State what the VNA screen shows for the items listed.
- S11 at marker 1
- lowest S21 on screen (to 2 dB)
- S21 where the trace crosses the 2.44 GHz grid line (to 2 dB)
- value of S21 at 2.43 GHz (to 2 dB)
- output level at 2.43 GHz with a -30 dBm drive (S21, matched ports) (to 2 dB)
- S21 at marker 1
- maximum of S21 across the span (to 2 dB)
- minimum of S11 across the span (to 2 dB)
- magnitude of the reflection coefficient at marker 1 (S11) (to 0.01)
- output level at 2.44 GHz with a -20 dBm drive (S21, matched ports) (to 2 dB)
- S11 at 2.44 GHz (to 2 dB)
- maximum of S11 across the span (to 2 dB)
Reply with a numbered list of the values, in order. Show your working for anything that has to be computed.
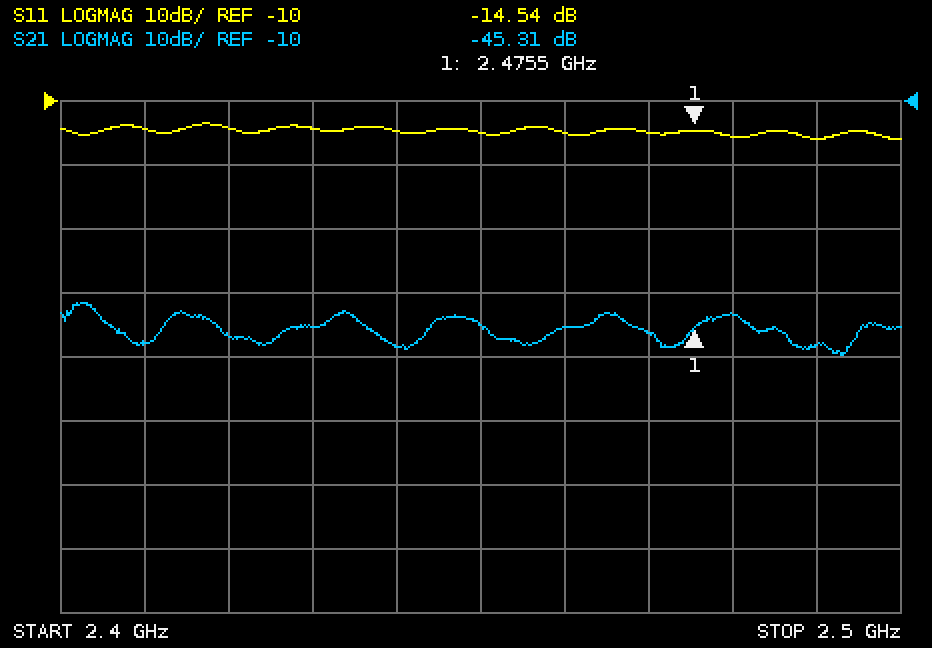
1. -14.54 dB
2. -50 dB
3. -48 dB
4. -46 dB
5. -30 dBm + (-46 dB) = -76 dBm
6. -45.31 dB
7. -42 dB
8. -16 dB
9. 10^(-14.54/20) ≈ 0.19
10. -20 dBm + (-48 dB) = -68 dBm
11. -14 dB
12. -14 dB
